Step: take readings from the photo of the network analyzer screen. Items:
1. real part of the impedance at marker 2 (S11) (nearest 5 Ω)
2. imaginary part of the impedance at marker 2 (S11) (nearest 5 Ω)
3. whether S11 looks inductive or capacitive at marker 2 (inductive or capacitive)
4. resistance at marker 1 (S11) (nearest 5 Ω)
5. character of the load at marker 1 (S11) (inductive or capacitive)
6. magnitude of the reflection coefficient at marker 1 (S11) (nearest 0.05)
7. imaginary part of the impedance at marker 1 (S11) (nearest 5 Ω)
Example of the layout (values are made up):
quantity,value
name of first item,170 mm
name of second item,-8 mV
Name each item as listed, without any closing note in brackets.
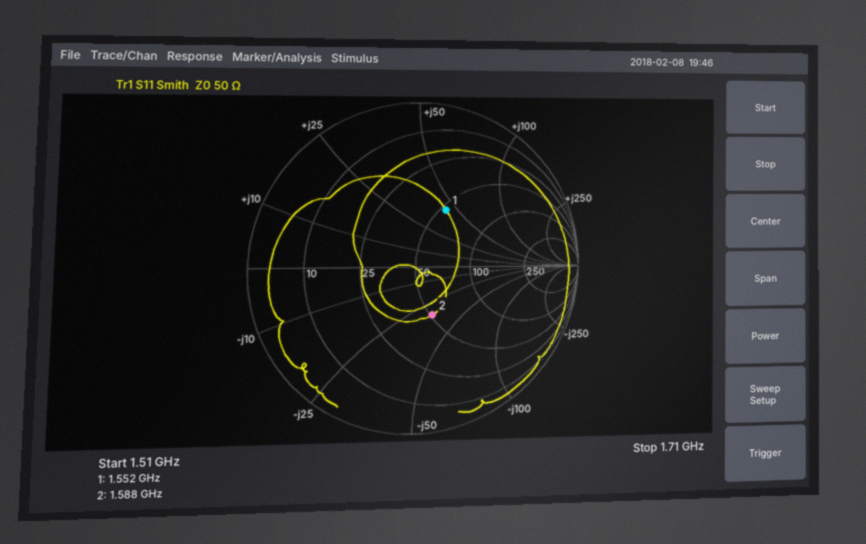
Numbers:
quantity,value
real part of the impedance at marker 2 (S11),50 Ω
imaginary part of the impedance at marker 2 (S11),-35 Ω
whether S11 looks inductive or capacitive at marker 2,capacitive
resistance at marker 1 (S11),55 Ω
character of the load at marker 1 (S11),inductive
magnitude of the reflection coefficient at marker 1 (S11),0.40
imaginary part of the impedance at marker 1 (S11),+45 Ω
